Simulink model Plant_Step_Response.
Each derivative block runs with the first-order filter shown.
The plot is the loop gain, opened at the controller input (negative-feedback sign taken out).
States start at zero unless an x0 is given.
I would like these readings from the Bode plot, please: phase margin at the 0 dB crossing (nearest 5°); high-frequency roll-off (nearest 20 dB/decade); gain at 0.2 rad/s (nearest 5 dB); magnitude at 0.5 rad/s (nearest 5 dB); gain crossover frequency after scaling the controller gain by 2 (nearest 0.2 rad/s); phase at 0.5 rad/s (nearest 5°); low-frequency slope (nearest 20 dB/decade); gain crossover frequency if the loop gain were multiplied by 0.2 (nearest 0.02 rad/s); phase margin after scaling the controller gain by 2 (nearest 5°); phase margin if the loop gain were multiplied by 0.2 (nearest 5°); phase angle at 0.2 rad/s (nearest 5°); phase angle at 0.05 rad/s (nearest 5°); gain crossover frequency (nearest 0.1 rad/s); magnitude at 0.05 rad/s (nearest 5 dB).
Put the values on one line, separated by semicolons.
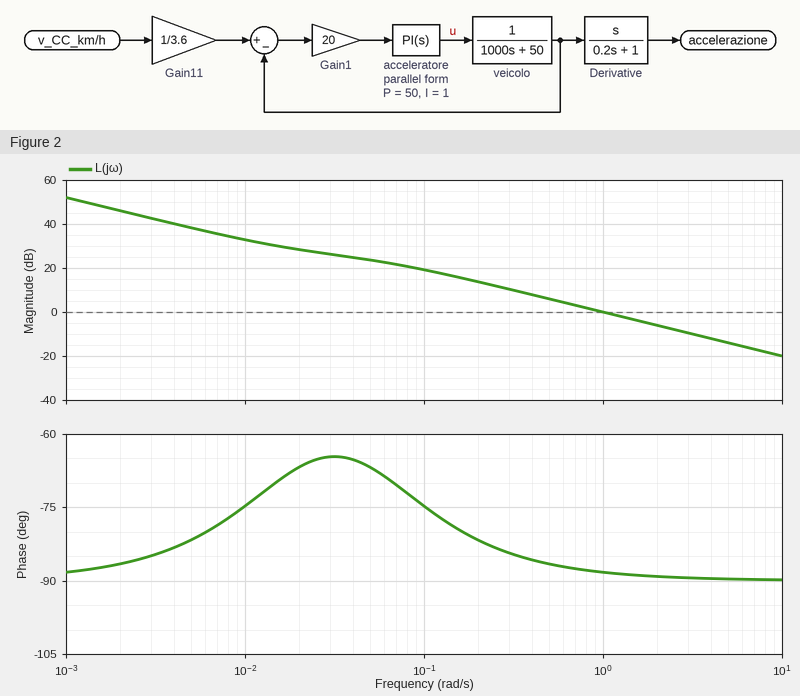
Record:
90°; -20 dB/decade; 15 dB; 5 dB; 2.0 rad/s; -85°; -20 dB/decade; 0.20 rad/s; 90°; 100°; -80°; -65°; 1.0 rad/s; 25 dB
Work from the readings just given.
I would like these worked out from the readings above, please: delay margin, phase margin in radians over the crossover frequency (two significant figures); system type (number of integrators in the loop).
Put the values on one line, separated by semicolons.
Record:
1.6 s; 1
